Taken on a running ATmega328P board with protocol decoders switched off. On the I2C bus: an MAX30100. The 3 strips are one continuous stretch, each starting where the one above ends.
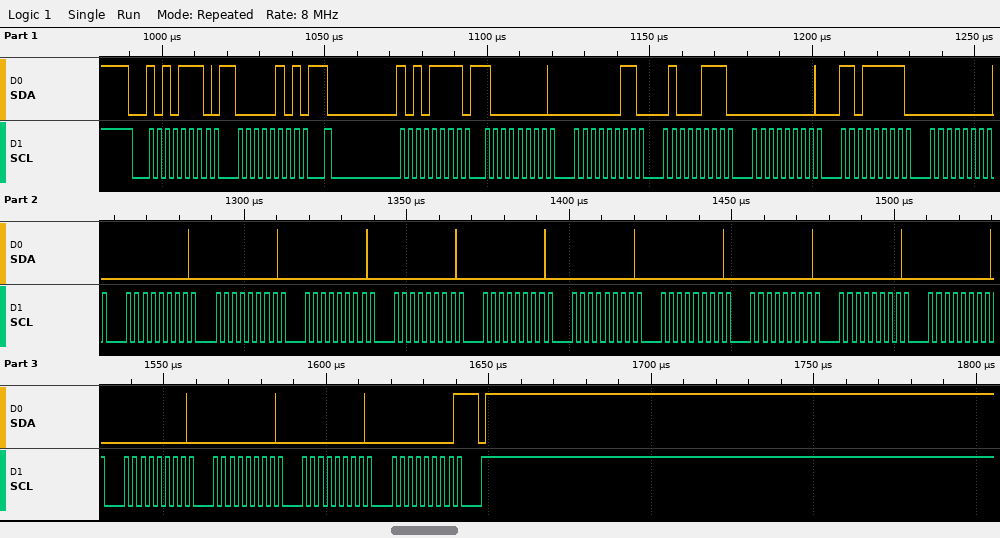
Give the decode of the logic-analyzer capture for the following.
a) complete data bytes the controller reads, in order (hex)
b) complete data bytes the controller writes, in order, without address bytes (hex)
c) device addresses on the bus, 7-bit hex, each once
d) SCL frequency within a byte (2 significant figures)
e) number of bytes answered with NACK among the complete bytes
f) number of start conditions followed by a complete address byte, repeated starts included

80 03 47 00 DF 00 00 00 00 00 00 00 00 00 00 00 00 00 00 00
05
0x57
400 kHz
1
2
